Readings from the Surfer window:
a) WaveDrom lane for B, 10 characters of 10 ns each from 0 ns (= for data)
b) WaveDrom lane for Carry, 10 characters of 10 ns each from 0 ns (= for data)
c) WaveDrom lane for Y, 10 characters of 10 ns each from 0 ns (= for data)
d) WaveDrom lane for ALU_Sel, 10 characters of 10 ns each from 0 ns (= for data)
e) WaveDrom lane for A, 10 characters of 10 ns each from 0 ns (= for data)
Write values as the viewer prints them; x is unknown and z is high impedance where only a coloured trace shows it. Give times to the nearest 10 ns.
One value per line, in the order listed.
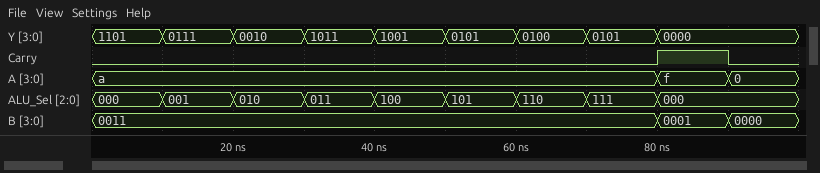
{name: 'B', wave: '=.......==', data: '0011 0001 0000'}
{name: 'Carry', wave: '0.......10'}
{name: 'Y', wave: '=========.', data: '1101 0111 0010 1011 1001 0101 0100 0101 0000'}
{name: 'ALU_Sel', wave: '=========.', data: '000 001 010 011 100 101 110 111 000'}
{name: 'A', wave: '=.......==', data: 'a f 0'}
